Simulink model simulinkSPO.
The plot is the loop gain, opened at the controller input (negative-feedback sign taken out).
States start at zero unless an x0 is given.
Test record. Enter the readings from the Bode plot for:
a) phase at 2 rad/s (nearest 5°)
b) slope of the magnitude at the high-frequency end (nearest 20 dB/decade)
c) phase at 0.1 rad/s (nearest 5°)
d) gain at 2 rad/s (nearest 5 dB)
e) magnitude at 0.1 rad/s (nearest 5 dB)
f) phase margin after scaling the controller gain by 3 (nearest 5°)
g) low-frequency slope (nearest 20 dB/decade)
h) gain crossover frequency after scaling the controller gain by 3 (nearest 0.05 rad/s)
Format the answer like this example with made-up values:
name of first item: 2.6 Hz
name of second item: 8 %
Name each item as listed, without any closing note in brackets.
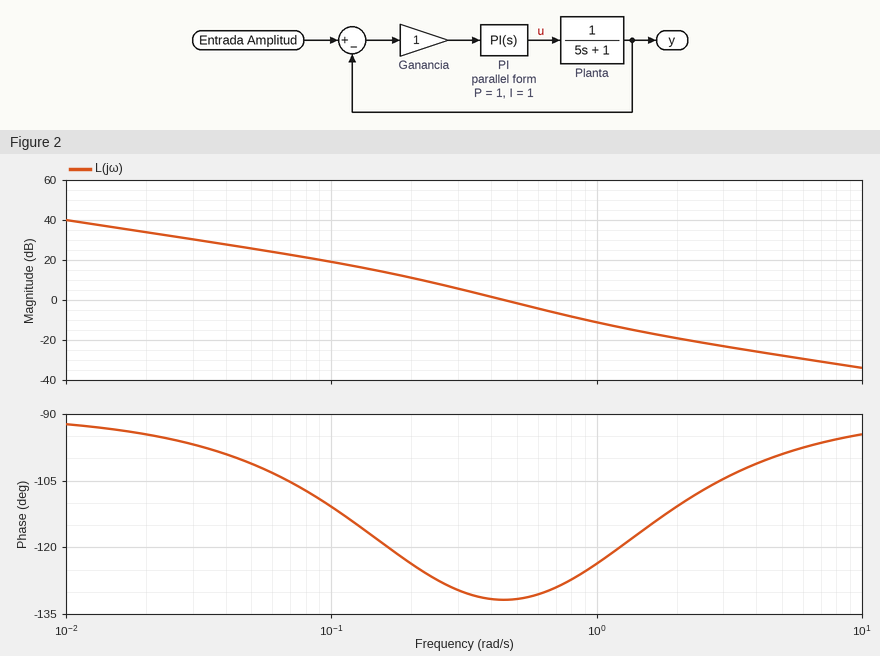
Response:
phase at 2 rad/s: -110°
slope of the magnitude at the high-frequency end: -20 dB/decade
phase at 0.1 rad/s: -110°
gain at 2 rad/s: -20 dB
magnitude at 0.1 rad/s: 20 dB
phase margin after scaling the controller gain by 3: 55°
low-frequency slope: -20 dB/decade
gain crossover frequency after scaling the controller gain by 3: 0.90 rad/s
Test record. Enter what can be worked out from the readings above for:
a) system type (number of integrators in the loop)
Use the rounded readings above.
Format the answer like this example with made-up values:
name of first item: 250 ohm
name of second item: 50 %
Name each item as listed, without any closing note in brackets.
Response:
system type: 1
